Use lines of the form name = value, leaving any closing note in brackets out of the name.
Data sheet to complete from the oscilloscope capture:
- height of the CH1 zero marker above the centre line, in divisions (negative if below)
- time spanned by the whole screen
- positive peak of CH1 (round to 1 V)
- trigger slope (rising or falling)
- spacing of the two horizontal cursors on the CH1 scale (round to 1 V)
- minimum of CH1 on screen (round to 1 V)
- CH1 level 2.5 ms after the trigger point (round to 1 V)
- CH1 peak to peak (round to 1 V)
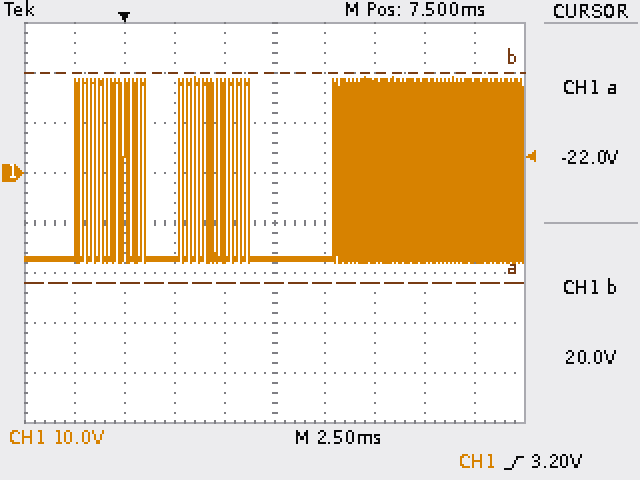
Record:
height of the CH1 zero marker above the centre line, in divisions = +1.0 div
time spanned by the whole screen = 25 ms
positive peak of CH1 = 19 V
trigger slope = rising
spacing of the two horizontal cursors on the CH1 scale = 42 V
minimum of CH1 on screen = -18 V
CH1 level 2.5 ms after the trigger point = -17 V
CH1 peak to peak = 37 V
